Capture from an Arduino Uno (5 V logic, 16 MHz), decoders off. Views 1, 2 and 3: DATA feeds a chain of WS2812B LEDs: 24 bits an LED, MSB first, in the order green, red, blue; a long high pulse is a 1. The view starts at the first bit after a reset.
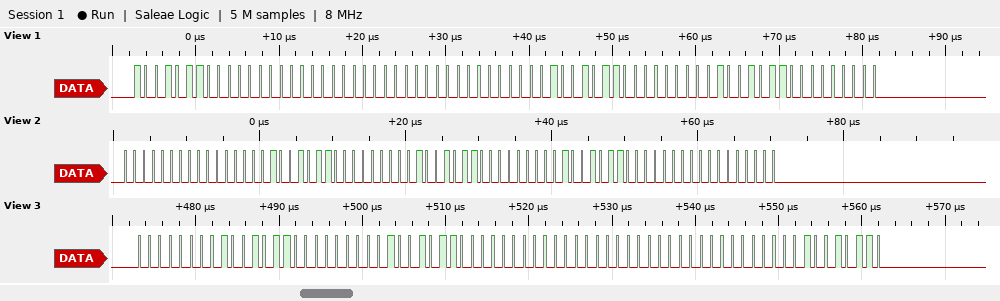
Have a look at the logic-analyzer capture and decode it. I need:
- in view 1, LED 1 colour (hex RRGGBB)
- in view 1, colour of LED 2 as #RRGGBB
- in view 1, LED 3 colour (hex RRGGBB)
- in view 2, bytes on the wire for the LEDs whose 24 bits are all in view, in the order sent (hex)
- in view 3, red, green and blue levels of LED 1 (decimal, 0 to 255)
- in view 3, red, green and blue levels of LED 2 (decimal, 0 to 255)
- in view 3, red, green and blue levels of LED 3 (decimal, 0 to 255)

#009600
#000096
#960000
00 00 96 00 96 00 96 00 00
150, 0, 0
0, 150, 0
0, 0, 150
